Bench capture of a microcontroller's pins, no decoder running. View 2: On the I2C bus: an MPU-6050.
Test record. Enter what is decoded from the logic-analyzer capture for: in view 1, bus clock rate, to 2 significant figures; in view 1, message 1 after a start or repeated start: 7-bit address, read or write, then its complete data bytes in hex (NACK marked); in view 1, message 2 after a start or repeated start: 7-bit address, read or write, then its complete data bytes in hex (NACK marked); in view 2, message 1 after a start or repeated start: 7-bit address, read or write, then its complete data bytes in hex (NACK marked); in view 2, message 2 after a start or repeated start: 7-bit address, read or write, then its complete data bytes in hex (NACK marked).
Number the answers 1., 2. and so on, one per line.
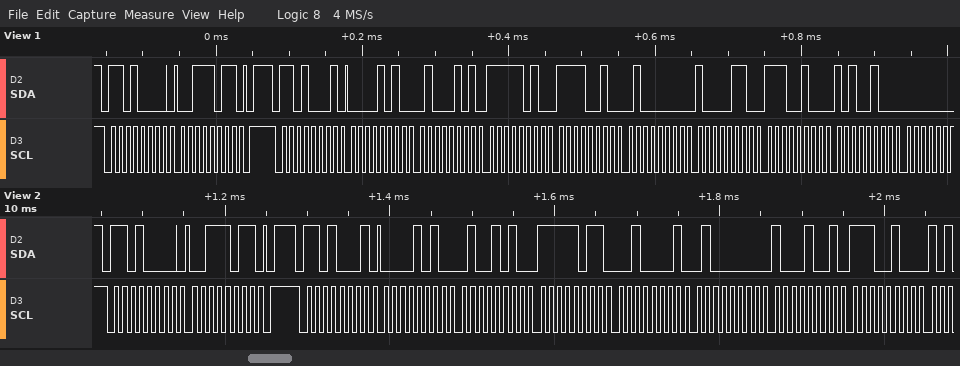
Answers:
1. 100 kHz
2. 0x68 write: 3B
3. 0x68 read: 0A 45 FA F2 40 86 E4 A4
4. 0x68 write: 3B
5. 0x68 read: 0A 4A FB 21 40 89 E4
